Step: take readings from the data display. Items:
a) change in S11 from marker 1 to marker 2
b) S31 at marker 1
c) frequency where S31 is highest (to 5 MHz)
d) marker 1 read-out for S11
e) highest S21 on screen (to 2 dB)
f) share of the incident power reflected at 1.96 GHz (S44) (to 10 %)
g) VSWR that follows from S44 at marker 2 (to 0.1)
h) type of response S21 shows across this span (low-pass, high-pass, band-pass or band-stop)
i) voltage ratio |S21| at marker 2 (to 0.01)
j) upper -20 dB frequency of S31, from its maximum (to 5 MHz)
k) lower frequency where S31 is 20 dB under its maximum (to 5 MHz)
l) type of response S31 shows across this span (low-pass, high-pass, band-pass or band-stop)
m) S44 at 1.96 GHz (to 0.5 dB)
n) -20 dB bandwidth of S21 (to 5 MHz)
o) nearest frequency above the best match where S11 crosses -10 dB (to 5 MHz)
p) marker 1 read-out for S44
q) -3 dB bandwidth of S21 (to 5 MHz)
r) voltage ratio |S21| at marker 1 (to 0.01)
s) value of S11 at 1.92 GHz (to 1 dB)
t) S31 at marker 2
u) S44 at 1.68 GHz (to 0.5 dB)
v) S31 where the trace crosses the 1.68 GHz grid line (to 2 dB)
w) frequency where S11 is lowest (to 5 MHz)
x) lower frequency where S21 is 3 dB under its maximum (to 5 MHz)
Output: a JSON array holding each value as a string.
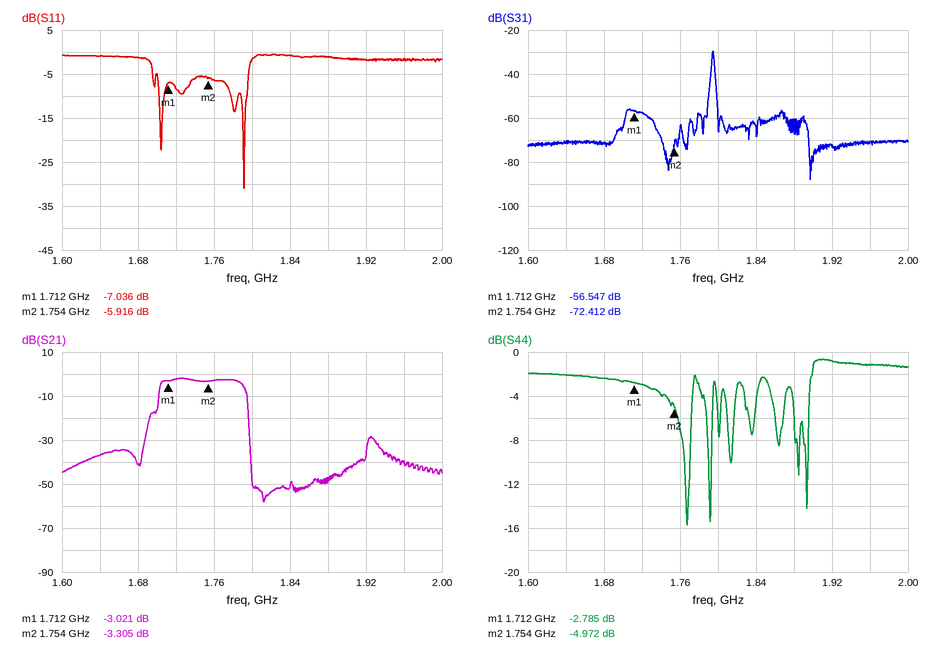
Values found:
["1.120 dB", "-56.547 dB", "1.795 GHz", "-7.036 dB", "-2 dB", "80 %", "3.6", "band-pass", "0.68", "1.800 GHz", "1.790 GHz", "band-pass", "-1.0 dB", "105 MHz", "1.795 GHz", "-2.785 dB", "85 MHz", "0.71", "-2 dB", "-72.412 dB", "-2.5 dB", "-72 dB", "1.790 GHz", "1.705 GHz"]
